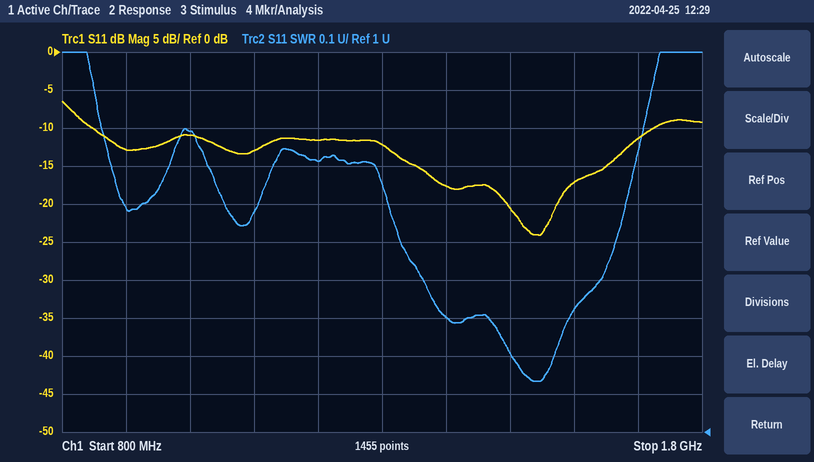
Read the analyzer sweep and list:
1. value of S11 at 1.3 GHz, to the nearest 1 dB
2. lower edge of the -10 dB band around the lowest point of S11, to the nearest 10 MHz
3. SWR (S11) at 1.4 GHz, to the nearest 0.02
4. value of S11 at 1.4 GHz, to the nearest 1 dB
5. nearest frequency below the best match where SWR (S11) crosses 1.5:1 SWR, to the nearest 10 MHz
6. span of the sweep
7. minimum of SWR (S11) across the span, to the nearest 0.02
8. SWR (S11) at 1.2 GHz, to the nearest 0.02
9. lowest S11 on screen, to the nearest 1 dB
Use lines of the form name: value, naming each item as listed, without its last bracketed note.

value of S11 at 1.3 GHz, to the nearest 1 dB: -12 dB
lower edge of the -10 dB band around the lowest point of S11, to the nearest 10 MHz: 850 MHz
SWR (S11) at 1.4 GHz, to the nearest 0.02: 1.30
value of S11 at 1.4 GHz, to the nearest 1 dB: -18 dB
nearest frequency below the best match where SWR (S11) crosses 1.5:1 SWR, to the nearest 10 MHz: 1.33 GHz
span of the sweep: 1 GHz
minimum of SWR (S11) across the span, to the nearest 0.02: 1.14
SWR (S11) at 1.2 GHz, to the nearest 0.02: 1.72
lowest S11 on screen, to the nearest 1 dB: -24 dB
